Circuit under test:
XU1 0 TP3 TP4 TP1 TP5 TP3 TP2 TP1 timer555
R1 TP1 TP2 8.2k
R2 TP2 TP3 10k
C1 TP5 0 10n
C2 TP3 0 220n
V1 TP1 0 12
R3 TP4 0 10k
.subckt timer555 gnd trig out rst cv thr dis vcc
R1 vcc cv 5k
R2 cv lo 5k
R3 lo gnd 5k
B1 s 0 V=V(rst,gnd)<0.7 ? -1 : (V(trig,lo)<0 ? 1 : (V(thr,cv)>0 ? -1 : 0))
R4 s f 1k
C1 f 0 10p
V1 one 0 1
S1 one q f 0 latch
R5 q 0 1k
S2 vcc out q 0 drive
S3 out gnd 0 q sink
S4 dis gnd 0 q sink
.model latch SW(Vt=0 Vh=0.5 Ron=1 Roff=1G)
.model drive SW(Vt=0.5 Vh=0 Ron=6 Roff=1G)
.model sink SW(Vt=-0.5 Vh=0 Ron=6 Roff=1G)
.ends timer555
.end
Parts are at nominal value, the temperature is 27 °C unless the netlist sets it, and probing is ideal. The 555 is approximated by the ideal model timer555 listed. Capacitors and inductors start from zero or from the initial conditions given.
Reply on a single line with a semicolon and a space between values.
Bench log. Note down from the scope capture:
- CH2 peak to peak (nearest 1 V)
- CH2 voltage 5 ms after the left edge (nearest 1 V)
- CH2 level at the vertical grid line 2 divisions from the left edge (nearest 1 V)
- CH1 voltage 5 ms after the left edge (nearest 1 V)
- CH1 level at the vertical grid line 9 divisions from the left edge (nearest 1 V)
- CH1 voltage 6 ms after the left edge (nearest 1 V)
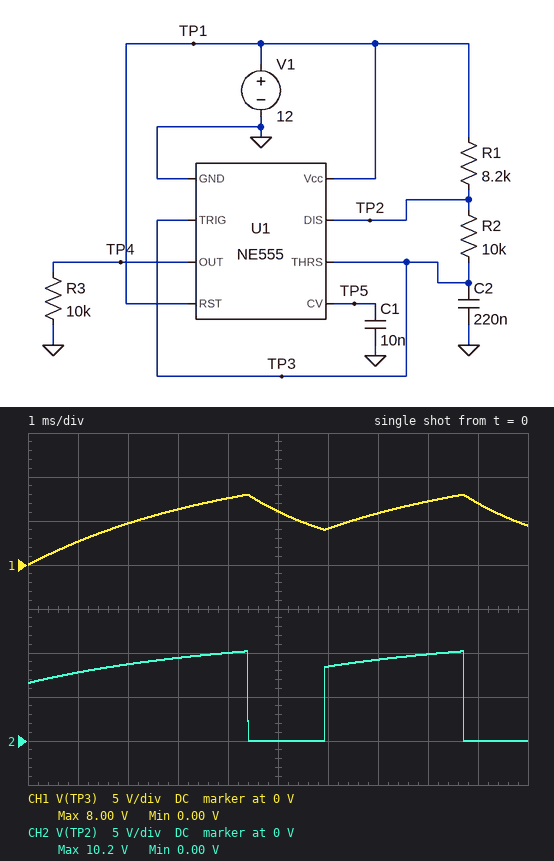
10 V; 0 V; 9 V; 6 V; 7 V; 4 V
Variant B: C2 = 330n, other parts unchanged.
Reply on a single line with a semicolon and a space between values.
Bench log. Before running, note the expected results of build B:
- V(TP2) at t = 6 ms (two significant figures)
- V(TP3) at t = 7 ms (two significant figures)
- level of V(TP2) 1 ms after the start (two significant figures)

10 V; 7.1 V; 7.4 V
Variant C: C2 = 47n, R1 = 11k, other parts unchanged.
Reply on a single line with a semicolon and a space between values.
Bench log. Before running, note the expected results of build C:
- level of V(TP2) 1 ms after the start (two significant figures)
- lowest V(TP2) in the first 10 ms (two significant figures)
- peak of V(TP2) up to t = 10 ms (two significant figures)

9.7 V; 8.9 mV; 9.9 V
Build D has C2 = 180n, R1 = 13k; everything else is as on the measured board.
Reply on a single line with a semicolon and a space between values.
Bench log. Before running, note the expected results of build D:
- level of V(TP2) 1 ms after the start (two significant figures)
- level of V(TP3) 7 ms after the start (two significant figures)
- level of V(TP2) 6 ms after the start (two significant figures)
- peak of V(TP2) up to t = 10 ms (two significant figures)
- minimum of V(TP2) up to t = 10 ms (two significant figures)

6.7 V; 6.0 V; 7.7 V; 9.7 V; 7.9 mV
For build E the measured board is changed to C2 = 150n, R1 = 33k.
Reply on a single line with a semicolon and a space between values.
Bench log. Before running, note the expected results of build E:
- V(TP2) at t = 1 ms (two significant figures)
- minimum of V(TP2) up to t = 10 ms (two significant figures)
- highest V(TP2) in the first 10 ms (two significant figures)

4.1 V; 4.6 mV; 8.9 V
